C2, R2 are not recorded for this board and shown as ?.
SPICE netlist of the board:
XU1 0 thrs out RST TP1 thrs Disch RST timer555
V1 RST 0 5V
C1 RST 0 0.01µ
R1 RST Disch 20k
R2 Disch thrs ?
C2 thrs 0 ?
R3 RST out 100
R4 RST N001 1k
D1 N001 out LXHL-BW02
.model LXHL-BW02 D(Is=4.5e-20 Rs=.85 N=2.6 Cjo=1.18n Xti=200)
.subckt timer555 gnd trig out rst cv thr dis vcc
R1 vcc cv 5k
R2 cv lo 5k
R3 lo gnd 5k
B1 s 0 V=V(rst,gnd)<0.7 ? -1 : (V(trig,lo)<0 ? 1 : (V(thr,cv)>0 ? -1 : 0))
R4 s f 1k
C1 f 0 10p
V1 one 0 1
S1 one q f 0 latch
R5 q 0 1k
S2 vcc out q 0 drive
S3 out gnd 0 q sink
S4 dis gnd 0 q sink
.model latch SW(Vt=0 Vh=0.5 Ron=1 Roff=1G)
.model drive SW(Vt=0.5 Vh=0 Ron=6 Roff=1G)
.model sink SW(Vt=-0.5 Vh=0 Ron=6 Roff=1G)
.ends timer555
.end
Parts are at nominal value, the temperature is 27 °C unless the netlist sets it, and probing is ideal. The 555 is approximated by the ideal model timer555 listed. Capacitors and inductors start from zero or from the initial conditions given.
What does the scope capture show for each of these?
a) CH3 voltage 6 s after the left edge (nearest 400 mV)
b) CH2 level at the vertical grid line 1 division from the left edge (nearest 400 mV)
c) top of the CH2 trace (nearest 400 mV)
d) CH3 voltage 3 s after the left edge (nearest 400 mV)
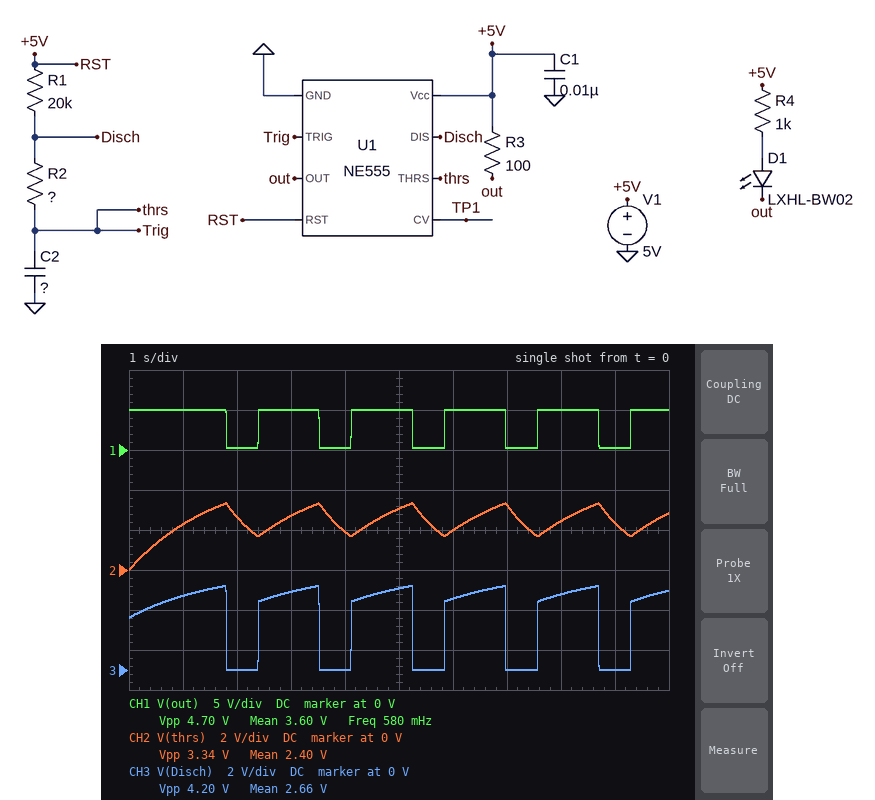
3.6 V
2.4 V
3.2 V
4.0 V
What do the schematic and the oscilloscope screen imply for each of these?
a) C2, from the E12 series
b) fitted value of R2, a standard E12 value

39 µF
22 kΩ
